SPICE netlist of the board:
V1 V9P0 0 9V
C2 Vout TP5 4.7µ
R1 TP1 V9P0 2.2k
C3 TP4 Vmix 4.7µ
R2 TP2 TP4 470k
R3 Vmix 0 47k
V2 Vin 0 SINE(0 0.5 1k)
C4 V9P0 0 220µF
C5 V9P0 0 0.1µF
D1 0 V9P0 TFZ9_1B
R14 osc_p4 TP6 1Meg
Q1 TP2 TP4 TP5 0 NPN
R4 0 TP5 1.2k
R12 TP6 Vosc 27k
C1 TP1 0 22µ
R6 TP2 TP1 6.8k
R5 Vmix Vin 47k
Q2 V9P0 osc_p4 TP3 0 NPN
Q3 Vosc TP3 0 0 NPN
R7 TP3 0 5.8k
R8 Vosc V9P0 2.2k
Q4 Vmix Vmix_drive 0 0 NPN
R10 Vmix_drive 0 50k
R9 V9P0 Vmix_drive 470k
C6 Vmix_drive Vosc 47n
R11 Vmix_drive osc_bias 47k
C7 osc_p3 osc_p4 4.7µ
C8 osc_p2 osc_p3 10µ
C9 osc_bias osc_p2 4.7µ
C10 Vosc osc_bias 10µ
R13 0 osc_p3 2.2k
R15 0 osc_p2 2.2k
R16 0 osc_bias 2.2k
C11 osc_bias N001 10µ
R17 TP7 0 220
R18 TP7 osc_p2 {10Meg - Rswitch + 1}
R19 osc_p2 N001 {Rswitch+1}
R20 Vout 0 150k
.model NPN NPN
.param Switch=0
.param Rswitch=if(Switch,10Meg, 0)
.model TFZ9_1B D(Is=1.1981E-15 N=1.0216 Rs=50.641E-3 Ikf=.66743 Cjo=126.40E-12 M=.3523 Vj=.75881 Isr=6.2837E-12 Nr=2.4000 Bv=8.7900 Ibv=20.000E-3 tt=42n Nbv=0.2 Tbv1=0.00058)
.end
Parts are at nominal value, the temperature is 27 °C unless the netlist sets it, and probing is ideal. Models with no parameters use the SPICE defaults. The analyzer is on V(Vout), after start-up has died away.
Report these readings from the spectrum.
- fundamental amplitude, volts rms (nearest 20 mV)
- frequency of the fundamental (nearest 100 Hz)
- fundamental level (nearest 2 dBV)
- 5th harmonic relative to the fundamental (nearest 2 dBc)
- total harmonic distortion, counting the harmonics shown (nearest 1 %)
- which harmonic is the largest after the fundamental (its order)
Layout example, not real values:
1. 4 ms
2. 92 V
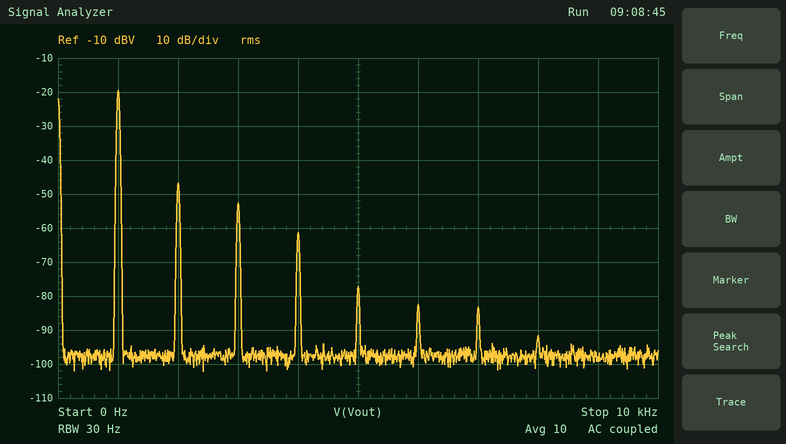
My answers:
1. 100 mV
2. 1.0 kHz
3. -20 dBV
4. -58 dBc
5. 5 %
6. 2
